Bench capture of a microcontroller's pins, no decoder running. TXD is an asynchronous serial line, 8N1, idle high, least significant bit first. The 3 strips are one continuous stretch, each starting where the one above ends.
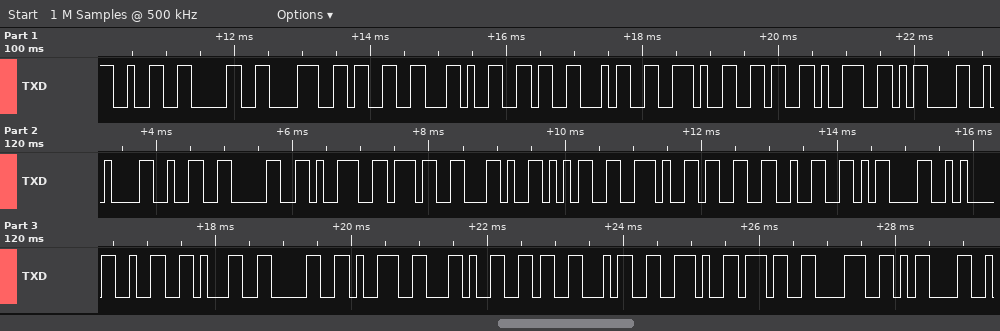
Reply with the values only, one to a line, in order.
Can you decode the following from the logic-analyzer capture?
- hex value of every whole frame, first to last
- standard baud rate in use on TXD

32 30 38 33 2C 36 34 2E 36 39 0D 0A 32 30 39 37 2C 35 2E 33 32 0D 0A 32 31 30 39 2C 36 34 2E 37 38 0D
9600 baud
